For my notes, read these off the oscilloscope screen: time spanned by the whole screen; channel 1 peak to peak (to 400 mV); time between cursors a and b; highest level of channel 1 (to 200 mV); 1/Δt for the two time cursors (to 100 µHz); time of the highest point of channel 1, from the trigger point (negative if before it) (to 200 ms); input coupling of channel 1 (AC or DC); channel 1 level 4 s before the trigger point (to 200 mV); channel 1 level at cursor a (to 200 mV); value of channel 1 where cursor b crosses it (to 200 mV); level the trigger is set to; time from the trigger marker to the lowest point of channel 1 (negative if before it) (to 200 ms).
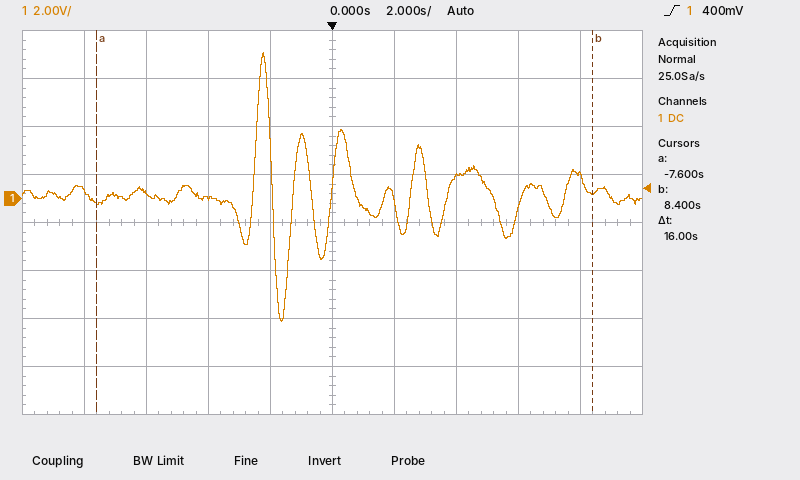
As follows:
20 s
11.2 V
16 s
6.0 V
62.5 mHz
-2.2 s
DC
0.0 V
-200 mV
200 mV
400 mV
-1.6 s
